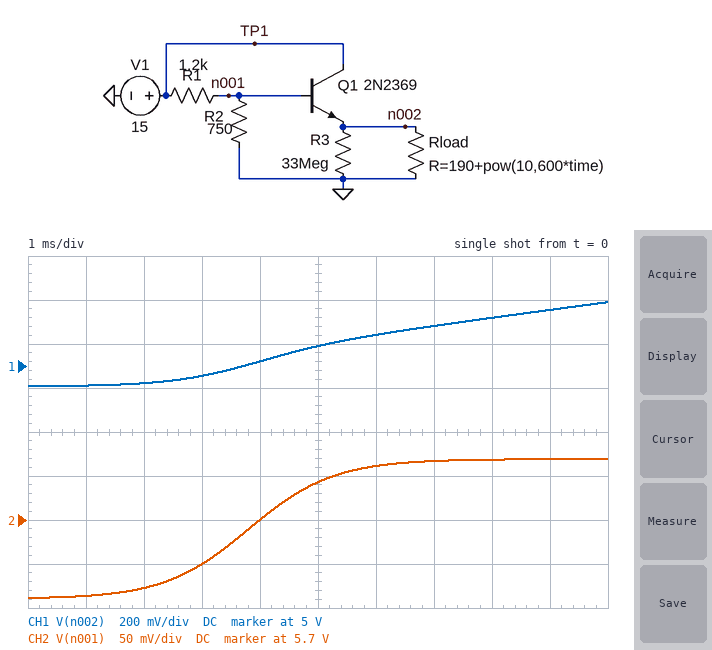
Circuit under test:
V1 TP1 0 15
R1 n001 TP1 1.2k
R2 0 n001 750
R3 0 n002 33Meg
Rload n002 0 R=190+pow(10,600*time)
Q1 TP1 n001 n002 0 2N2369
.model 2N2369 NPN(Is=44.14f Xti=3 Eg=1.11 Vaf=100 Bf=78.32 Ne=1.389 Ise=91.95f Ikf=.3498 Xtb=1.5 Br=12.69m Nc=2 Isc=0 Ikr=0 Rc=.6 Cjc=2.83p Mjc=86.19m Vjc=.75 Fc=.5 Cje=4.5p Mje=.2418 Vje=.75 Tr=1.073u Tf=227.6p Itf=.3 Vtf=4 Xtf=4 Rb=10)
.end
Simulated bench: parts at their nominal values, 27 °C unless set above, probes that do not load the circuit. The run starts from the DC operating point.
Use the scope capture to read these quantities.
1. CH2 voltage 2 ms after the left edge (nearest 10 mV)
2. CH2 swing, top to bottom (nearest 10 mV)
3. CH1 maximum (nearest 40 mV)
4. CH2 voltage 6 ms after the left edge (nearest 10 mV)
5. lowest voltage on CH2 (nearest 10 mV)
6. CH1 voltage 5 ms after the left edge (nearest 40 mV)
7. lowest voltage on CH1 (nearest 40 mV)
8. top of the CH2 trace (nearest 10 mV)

5.62 V
160 mV
5.28 V
5.76 V
5.61 V
5.08 V
4.92 V
5.77 V
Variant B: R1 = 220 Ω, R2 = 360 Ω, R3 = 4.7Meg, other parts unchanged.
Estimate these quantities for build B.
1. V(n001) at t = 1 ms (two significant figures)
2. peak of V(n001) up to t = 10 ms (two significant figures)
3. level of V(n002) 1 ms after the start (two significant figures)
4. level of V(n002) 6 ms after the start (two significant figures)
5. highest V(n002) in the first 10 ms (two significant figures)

9.2 V
9.3 V
8.5 V
8.7 V
8.8 V
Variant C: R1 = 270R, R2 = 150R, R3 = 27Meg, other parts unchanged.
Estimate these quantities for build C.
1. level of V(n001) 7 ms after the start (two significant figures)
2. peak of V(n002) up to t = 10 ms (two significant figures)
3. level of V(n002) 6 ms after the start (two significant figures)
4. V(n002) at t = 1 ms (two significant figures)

5.4 V
4.9 V
4.7 V
4.6 V
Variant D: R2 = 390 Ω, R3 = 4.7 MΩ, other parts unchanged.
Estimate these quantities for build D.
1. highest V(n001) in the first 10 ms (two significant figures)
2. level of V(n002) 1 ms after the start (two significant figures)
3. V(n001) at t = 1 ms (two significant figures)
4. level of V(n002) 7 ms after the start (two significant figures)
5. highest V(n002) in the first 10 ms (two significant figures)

3.7 V
2.9 V
3.6 V
3.1 V
3.2 V
